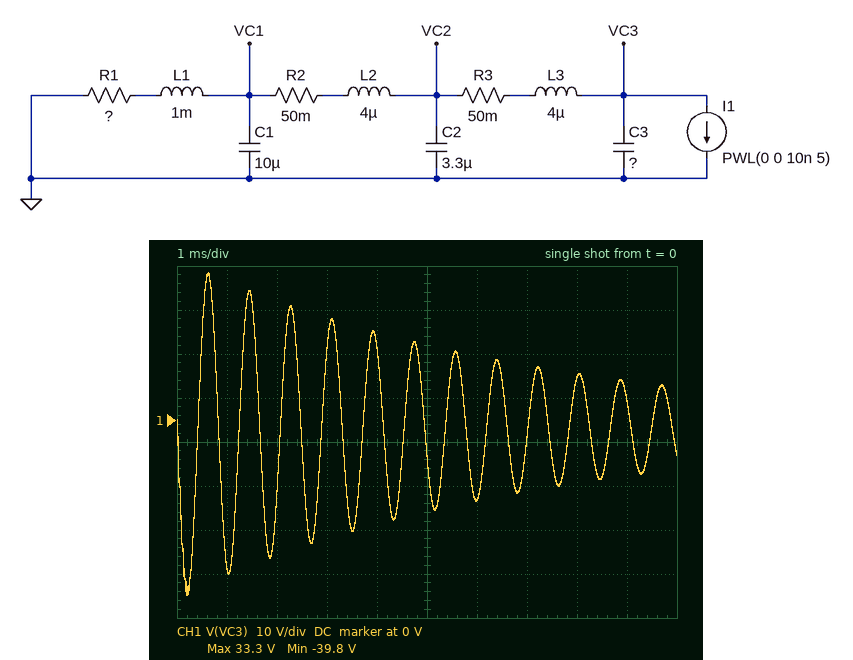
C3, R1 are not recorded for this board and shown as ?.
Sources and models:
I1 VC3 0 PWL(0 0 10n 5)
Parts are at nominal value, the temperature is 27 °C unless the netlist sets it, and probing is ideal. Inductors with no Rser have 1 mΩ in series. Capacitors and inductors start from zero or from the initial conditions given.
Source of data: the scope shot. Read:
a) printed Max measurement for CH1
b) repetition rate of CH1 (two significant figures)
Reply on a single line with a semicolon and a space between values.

33.3 V; 1.2 kHz
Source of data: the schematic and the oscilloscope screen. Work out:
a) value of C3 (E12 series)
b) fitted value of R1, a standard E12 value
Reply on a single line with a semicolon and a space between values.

3.9 µF; 0.27 Ω
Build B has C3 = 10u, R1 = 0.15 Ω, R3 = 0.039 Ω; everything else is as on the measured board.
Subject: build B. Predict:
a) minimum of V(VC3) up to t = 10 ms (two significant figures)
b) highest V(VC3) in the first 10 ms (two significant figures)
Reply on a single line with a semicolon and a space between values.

-34 V; 30 V
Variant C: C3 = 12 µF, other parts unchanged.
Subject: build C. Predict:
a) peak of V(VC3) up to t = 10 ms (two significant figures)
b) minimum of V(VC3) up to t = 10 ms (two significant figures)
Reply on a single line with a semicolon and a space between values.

26 V; -32 V
